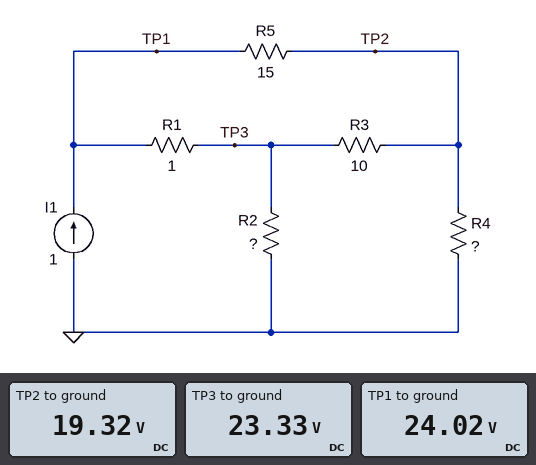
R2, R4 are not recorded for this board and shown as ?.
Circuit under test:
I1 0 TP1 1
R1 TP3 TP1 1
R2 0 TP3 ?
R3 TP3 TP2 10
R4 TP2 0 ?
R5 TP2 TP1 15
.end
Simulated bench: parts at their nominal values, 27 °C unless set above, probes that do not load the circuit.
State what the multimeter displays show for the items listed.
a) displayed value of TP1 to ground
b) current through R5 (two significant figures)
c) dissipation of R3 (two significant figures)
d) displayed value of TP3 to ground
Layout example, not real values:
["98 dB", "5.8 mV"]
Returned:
["24.02 V", "310 mA", "1.6 W", "23.33 V"]
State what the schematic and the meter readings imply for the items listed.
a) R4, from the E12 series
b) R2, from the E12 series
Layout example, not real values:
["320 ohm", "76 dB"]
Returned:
["27 Ω", "82 Ω"]
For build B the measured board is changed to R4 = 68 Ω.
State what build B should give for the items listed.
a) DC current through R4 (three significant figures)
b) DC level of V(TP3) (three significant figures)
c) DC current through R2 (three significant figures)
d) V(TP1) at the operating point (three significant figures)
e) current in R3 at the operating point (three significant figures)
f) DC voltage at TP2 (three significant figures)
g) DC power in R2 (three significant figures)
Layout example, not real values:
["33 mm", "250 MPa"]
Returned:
["528 mA", "38.7 V", "472 mA", "39.5 V", "286 mA", "35.9 V", "18.3 W"]
